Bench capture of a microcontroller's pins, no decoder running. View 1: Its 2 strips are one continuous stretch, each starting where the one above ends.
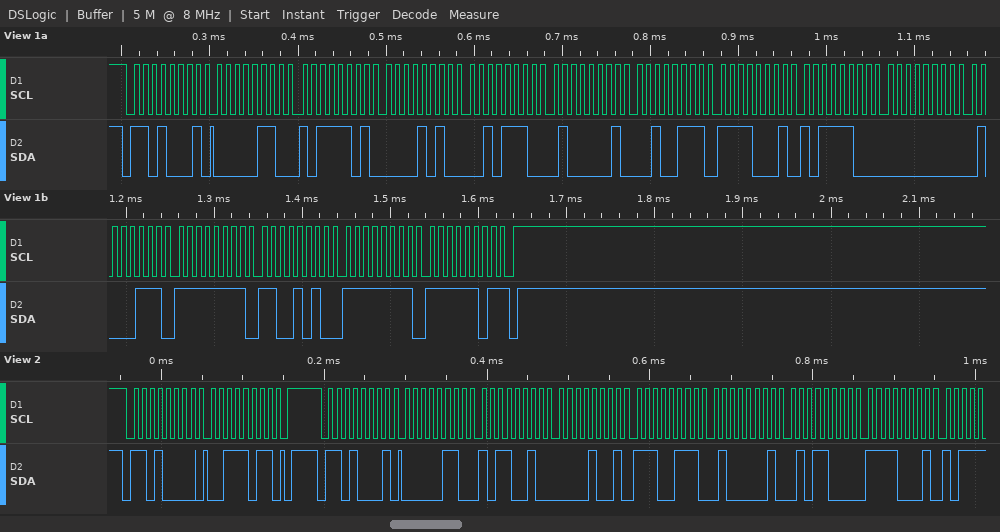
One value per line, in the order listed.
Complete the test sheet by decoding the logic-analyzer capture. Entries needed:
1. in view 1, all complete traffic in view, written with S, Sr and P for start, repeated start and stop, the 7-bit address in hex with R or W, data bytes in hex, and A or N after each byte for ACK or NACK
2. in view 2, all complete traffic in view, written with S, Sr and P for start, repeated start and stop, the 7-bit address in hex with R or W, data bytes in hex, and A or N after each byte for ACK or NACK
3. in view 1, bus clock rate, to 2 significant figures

S 68R A 06 A BD A 0A A 2E A 41 A 27 A F1 A BC A 00 A 47 A FF A CA A FF A FD N P
S 68W A 3B A P S 68R A 06 A B2 A 09 A E7 A 41 A 58 A F1 A
100 kHz
